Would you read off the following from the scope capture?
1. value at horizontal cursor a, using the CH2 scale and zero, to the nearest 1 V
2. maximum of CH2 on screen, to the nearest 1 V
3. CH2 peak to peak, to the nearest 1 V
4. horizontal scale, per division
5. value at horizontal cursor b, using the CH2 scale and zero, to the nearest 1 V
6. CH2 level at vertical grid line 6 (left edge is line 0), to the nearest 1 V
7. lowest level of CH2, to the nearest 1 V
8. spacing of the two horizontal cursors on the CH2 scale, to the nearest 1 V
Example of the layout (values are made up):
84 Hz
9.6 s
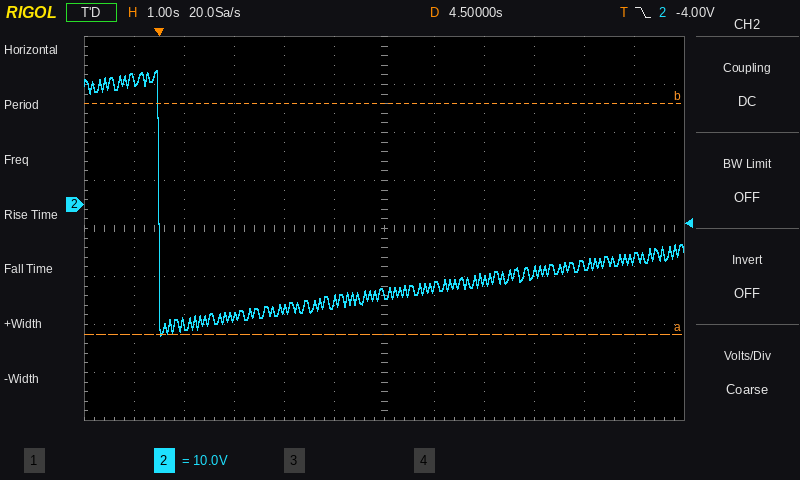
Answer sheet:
-27 V
28 V
55 V
1 s
21 V
-19 V
-27 V
48 V
